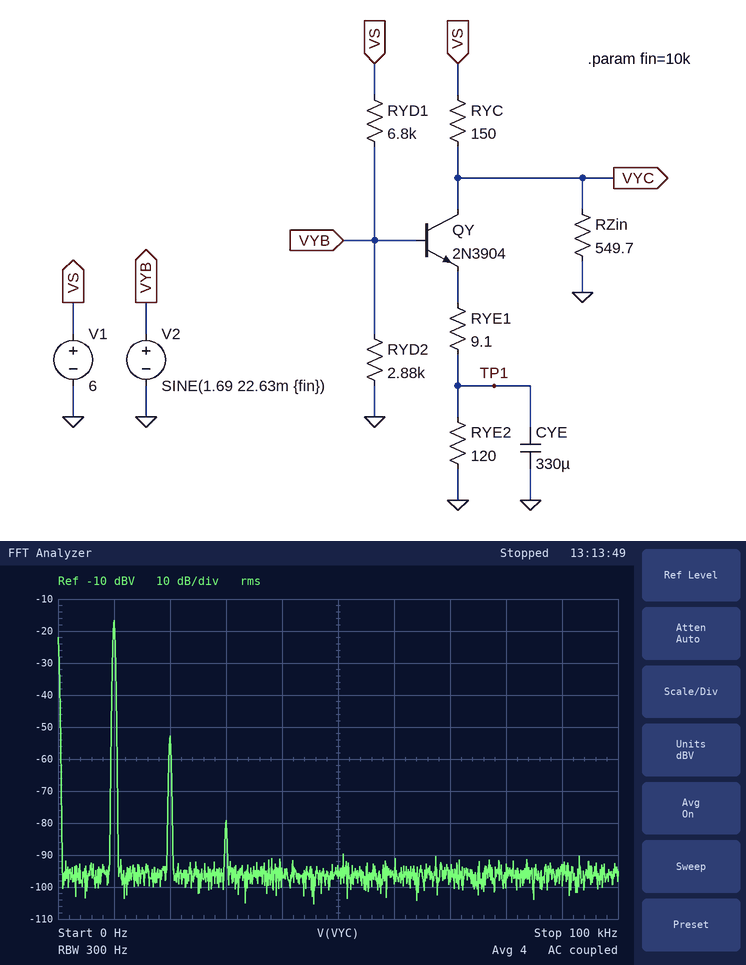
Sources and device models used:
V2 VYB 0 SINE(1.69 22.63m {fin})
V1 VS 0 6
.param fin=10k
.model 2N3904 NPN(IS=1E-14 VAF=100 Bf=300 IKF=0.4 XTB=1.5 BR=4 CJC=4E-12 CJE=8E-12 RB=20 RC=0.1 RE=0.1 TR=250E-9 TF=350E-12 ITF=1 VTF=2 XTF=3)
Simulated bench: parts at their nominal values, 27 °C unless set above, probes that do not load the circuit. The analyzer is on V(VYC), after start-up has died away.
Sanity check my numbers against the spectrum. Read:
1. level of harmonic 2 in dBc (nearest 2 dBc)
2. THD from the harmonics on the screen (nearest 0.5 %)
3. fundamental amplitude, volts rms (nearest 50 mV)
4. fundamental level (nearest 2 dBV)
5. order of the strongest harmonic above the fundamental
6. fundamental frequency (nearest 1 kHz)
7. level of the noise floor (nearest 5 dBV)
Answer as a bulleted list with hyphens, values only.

- -36 dBc
- 1.5 %
- 150 mV
- -16 dBV
- 2
- 10 kHz
- -95 dBV
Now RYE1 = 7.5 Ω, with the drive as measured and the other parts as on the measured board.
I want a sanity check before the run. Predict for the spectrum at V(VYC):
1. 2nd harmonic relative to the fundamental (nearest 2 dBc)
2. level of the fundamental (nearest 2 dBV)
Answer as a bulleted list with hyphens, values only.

- -34 dBc
- -16 dBV
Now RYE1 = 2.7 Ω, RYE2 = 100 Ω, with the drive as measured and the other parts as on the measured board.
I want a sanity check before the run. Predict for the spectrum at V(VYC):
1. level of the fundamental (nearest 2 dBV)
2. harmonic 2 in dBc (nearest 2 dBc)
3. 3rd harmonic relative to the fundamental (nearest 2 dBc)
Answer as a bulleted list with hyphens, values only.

- -10 dBV
- -26 dBc
- -54 dBc
